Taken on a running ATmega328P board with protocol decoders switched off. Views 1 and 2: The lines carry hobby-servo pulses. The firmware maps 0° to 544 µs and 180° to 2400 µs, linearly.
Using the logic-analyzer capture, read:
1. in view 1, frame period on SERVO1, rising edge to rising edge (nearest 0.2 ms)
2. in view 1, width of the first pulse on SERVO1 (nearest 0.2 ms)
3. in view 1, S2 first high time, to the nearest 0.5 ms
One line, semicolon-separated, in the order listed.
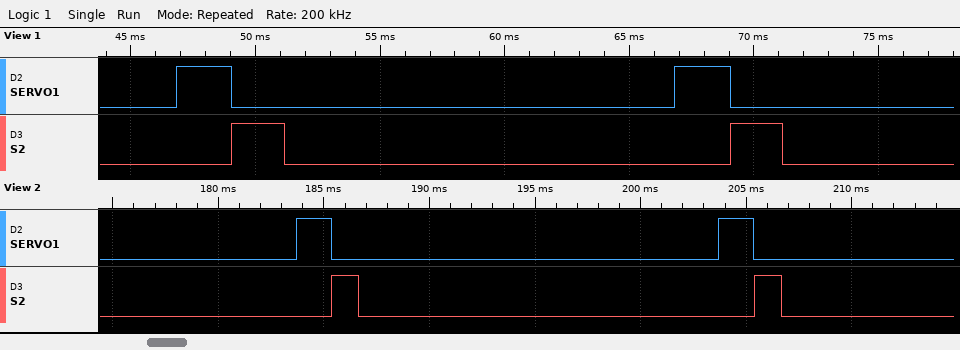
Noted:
20.0 ms; 2.2 ms; 2.0 ms
